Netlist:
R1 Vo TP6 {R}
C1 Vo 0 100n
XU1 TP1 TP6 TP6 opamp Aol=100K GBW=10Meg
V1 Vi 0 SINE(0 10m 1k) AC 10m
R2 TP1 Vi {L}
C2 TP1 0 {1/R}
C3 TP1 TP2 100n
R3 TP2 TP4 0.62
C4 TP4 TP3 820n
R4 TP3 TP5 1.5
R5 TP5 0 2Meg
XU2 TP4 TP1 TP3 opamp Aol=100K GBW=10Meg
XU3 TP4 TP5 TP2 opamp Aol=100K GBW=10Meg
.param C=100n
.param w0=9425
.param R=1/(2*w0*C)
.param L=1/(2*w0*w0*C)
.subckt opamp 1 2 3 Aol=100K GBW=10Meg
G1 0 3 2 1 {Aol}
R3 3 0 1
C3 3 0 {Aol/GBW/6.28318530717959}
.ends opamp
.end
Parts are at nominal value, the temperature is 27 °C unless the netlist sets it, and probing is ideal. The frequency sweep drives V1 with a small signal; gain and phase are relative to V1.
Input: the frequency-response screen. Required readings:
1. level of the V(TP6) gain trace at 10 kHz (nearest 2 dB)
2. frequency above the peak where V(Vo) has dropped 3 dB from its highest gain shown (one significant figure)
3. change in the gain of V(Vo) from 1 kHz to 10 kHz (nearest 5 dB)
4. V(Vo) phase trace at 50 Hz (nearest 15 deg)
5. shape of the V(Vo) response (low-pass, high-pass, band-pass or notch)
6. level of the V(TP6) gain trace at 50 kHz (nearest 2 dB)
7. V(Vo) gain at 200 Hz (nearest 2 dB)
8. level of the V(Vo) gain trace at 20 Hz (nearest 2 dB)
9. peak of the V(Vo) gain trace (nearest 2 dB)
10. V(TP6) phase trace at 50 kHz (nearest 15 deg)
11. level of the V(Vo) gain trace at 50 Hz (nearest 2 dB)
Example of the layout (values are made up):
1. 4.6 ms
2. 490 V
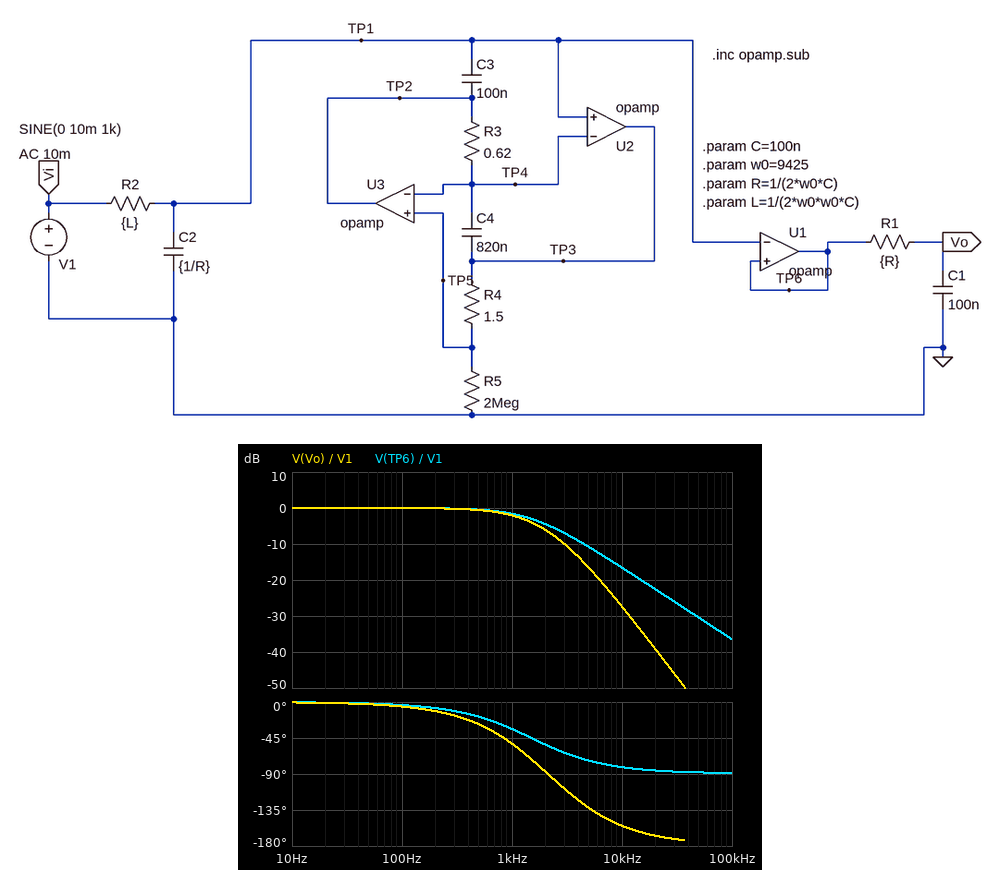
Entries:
1. -16 dB
2. 1 kHz
3. -25 dB
4. 0 deg
5. low-pass
6. -30 dB
7. 0 dB
8. 0 dB
9. 0 dB
10. -90 deg
11. 0 dB
